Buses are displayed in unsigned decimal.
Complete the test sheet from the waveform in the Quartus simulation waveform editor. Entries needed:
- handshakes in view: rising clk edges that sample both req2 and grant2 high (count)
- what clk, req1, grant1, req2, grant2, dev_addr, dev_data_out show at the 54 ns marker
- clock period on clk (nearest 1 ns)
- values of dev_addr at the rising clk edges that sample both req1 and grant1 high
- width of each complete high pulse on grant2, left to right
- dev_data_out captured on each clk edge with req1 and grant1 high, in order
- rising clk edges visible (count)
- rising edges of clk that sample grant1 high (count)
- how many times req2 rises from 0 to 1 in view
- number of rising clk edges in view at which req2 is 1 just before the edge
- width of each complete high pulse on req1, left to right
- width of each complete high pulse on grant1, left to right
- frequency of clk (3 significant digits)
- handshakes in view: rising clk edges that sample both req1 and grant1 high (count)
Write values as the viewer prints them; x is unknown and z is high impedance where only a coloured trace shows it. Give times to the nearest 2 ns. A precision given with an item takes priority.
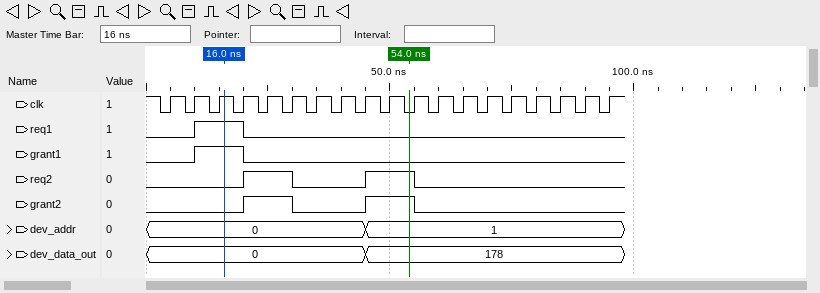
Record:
4
clk=0, req1=0, grant1=0, req2=1, grant2=1, dev_addr=1, dev_data_out=178
5 ns
0, 0
10 ns, 10 ns
0, 0
19
2
2
4
10 ns
10 ns
200 MHz
2
